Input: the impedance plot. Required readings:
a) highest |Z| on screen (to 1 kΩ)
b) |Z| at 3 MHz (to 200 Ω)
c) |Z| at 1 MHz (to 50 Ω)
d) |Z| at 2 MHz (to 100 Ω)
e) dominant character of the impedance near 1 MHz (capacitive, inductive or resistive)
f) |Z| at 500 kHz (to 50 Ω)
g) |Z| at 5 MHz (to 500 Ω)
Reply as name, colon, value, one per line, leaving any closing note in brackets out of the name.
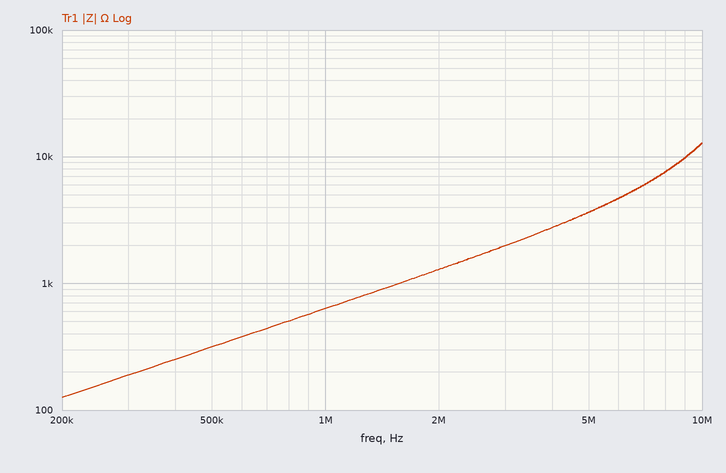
highest |Z| on screen: 13 kΩ
|Z| at 3 MHz: 2.0 kΩ
|Z| at 1 MHz: 650 Ω
|Z| at 2 MHz: 1.3 kΩ
dominant character of the impedance near 1 MHz: inductive
|Z| at 500 kHz: 300 Ω
|Z| at 5 MHz: 3.5 kΩ
